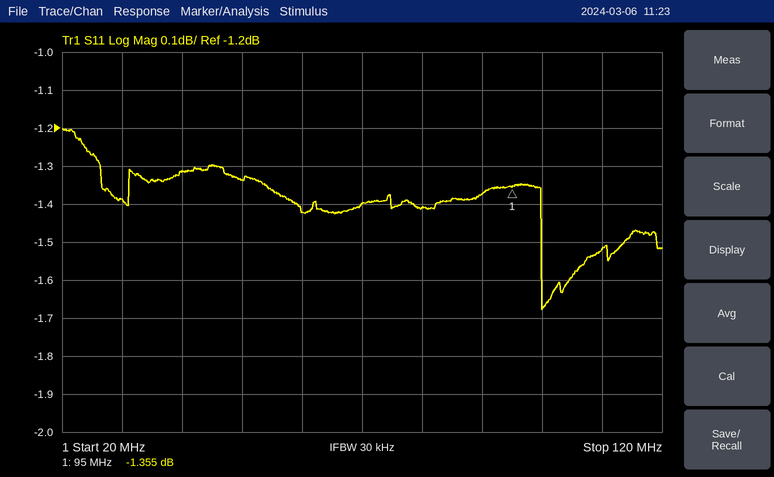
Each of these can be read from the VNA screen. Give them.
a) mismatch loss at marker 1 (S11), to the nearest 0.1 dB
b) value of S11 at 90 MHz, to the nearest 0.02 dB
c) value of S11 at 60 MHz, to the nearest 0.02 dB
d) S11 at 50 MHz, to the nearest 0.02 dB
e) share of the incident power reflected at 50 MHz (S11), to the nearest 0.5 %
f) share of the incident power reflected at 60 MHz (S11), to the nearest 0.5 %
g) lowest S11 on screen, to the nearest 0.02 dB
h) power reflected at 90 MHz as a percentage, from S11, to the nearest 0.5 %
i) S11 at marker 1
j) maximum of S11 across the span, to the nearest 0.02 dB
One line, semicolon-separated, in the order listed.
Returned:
5.7 dB; -1.38 dB; -1.42 dB; -1.34 dB; 73.5 %; 72.0 %; -1.68 dB; 73.0 %; -1.355 dB; -1.20 dB
